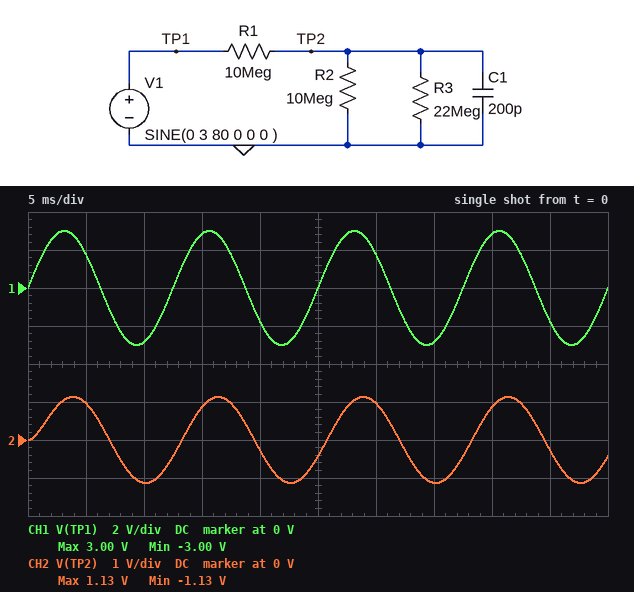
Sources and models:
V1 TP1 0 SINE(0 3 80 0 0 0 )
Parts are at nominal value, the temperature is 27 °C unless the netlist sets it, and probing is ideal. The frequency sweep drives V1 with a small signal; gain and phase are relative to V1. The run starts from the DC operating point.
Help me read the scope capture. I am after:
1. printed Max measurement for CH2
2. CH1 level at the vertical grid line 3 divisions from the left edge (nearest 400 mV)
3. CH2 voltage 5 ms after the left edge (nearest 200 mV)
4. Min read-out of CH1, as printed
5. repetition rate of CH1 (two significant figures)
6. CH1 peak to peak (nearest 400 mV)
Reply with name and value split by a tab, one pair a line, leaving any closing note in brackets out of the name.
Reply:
printed Max measurement for CH2	1.13 V
CH1 level at the vertical grid line 3 divisions from the left edge	2.8 V
CH2 voltage 5 ms after the left edge	1.0 V
Min read-out of CH1, as printed	-3.00 V
repetition rate of CH1	80 Hz
CH1 peak to peak	6.0 V
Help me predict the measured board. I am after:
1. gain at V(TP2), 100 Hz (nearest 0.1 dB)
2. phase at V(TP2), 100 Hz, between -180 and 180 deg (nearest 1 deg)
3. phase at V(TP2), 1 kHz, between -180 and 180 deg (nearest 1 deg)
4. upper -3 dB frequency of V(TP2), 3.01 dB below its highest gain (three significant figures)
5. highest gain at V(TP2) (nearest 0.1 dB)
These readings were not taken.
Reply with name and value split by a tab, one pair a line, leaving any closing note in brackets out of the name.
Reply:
gain at V(TP2), 100 Hz	-8.8 dB
phase at V(TP2), 100 Hz, between -180 and 180 deg	-27 deg
phase at V(TP2), 1 kHz, between -180 and 180 deg	-79 deg
upper -3 dB frequency of V(TP2), 3.01 dB below its highest gain	195 Hz
highest gain at V(TP2)	-7.8 dB
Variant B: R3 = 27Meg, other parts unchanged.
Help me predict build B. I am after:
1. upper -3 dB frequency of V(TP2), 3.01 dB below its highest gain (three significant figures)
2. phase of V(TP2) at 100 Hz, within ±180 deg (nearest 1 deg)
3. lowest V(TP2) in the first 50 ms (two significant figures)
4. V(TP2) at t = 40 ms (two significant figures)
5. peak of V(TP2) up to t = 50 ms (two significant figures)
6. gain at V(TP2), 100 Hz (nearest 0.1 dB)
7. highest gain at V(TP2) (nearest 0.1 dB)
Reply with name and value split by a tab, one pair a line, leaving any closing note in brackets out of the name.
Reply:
upper -3 dB frequency of V(TP2), 3.01 dB below its highest gain	189 Hz
phase of V(TP2) at 100 Hz, within ±180 deg	-28 deg
lowest V(TP2) in the first 50 ms	-1.2 V
V(TP2) at t = 40 ms	880 mV
peak of V(TP2) up to t = 50 ms	1.2 V
gain at V(TP2), 100 Hz	-8.6 dB
highest gain at V(TP2)	-7.5 dB
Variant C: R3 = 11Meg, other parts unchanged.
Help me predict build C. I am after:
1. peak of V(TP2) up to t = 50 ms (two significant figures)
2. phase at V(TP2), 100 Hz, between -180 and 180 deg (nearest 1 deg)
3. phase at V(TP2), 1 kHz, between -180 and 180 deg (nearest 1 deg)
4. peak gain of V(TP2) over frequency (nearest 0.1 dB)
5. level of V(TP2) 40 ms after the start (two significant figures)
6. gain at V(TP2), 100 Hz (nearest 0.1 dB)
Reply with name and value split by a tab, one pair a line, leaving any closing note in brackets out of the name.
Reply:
peak of V(TP2) up to t = 50 ms	980 mV
phase at V(TP2), 100 Hz, between -180 and 180 deg	-23 deg
phase at V(TP2), 1 kHz, between -180 and 180 deg	-77 deg
peak gain of V(TP2) over frequency	-9.3 dB
level of V(TP2) 40 ms after the start	780 mV
gain at V(TP2), 100 Hz	-10.0 dB
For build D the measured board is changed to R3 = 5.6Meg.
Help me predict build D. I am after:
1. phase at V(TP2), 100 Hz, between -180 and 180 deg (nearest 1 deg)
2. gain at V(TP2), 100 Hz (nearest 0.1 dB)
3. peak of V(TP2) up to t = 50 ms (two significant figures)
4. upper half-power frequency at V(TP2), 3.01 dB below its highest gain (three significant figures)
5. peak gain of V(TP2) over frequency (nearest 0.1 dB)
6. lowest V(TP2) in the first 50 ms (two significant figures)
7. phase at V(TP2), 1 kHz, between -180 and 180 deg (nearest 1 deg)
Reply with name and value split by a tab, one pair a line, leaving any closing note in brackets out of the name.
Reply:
phase at V(TP2), 100 Hz, between -180 and 180 deg	-18 deg
gain at V(TP2), 100 Hz	-12.0 dB
peak of V(TP2) up to t = 50 ms	770 mV
upper half-power frequency at V(TP2), 3.01 dB below its highest gain	301 Hz
peak gain of V(TP2) over frequency	-11.6 dB
lowest V(TP2) in the first 50 ms	-770 mV
phase at V(TP2), 1 kHz, between -180 and 180 deg	-73 deg
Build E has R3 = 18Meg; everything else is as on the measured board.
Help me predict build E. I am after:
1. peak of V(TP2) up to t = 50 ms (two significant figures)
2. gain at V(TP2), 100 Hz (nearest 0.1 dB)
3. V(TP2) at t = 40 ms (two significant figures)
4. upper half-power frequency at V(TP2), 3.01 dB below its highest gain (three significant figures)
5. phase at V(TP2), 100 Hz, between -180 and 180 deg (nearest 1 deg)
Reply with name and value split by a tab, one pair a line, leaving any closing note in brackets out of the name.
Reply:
peak of V(TP2) up to t = 50 ms	1.1 V
gain at V(TP2), 100 Hz	-9.1 dB
V(TP2) at t = 40 ms	840 mV
upper half-power frequency at V(TP2), 3.01 dB below its highest gain	203 Hz
phase at V(TP2), 100 Hz, between -180 and 180 deg	-26 deg
